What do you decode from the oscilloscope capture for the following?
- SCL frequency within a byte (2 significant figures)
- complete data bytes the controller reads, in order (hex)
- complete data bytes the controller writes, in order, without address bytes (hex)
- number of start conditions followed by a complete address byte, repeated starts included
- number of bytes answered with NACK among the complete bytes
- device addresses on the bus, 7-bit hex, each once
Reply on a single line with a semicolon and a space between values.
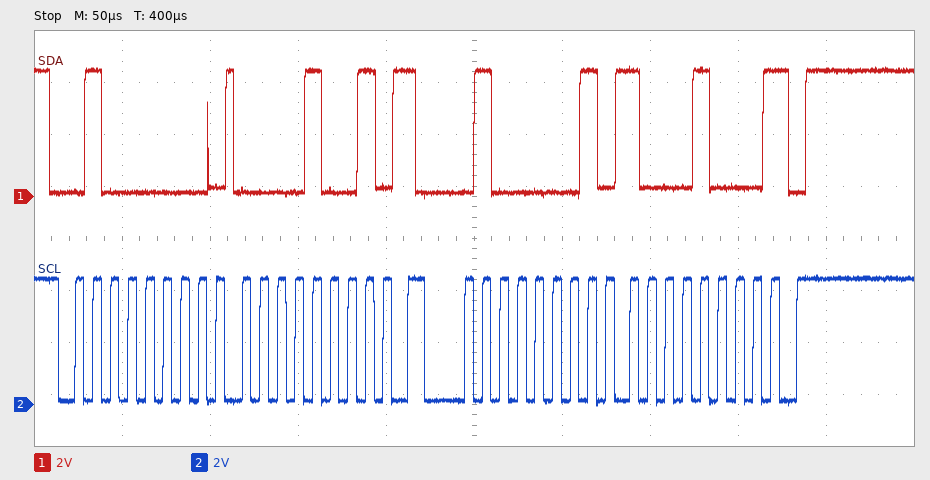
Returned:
100 kHz; 88; 09; 2; 1; 0x20
